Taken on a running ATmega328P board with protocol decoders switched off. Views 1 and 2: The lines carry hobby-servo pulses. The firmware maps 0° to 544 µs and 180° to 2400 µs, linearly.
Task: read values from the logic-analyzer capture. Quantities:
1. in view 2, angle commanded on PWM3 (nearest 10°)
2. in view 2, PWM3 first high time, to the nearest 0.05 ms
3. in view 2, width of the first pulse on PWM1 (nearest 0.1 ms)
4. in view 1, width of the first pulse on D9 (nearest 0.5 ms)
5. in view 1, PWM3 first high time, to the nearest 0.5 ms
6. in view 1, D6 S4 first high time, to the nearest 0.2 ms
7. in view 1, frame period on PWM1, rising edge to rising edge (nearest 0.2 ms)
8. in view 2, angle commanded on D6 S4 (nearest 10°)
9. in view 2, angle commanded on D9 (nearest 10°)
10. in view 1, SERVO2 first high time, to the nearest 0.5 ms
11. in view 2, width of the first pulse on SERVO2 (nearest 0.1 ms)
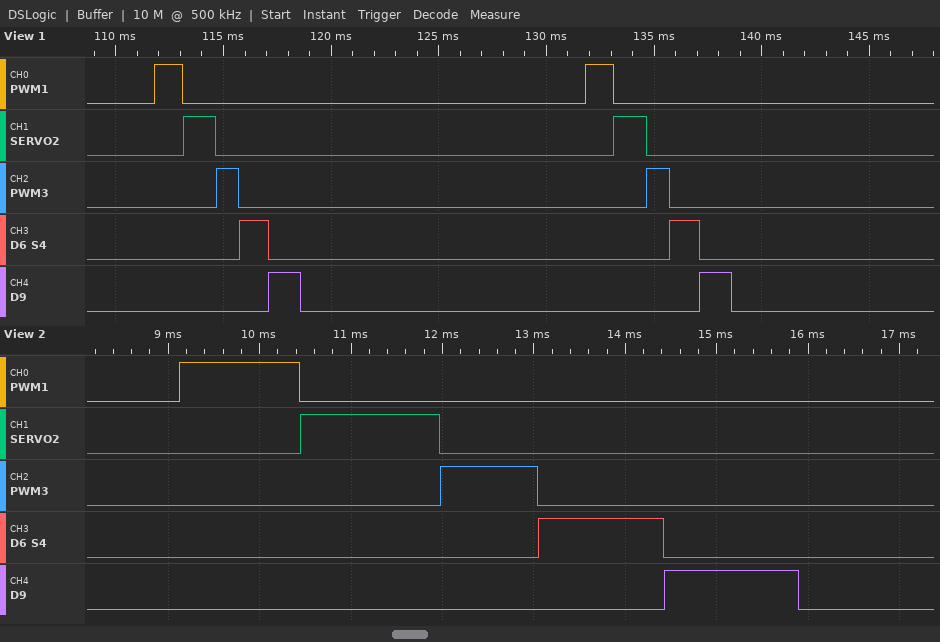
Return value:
50°
1.05 ms
1.3 ms
1.5 ms
1.0 ms
1.4 ms
20.0 ms
80°
90°
1.5 ms
1.5 ms
